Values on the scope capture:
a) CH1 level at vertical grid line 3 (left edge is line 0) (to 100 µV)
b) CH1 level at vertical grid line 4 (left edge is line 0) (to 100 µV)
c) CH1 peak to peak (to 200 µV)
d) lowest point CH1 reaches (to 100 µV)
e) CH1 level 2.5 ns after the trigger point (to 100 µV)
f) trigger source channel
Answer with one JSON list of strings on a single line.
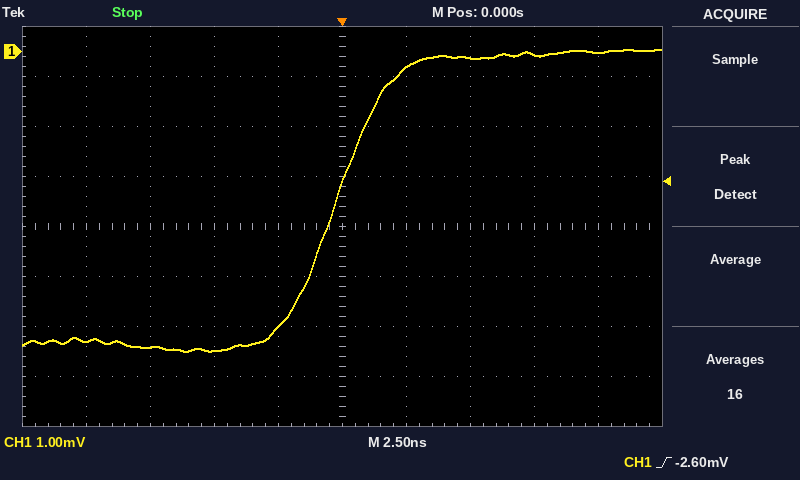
["-6.0 mV", "-5.5 mV", "6.0 mV", "-6.0 mV", "-300 µV", "CH1"]
